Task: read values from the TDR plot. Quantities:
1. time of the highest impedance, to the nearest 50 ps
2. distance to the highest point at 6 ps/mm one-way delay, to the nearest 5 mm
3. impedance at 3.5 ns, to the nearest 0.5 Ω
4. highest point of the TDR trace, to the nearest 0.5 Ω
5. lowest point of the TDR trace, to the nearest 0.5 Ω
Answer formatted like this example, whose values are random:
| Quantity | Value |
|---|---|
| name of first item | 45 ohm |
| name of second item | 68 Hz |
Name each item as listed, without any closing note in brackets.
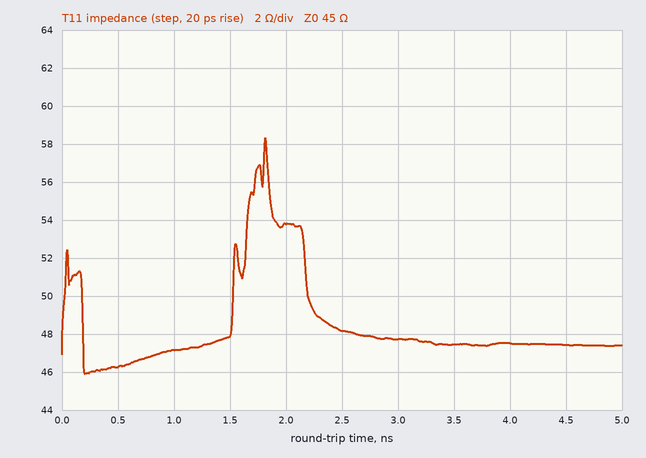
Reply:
| Quantity | Value |
|---|---|
| time of the highest impedance, to the nearest 50 ps | 1.80 ns |
| distance to the highest point at 6 ps/mm one-way delay, to the nearest 5 mm | 150 mm |
| impedance at 3.5 ns, to the nearest 0.5 Ω | 47.5 Ω |
| highest point of the TDR trace, to the nearest 0.5 Ω | 58.5 Ω |
| lowest point of the TDR trace, to the nearest 0.5 Ω | 46.0 Ω |
